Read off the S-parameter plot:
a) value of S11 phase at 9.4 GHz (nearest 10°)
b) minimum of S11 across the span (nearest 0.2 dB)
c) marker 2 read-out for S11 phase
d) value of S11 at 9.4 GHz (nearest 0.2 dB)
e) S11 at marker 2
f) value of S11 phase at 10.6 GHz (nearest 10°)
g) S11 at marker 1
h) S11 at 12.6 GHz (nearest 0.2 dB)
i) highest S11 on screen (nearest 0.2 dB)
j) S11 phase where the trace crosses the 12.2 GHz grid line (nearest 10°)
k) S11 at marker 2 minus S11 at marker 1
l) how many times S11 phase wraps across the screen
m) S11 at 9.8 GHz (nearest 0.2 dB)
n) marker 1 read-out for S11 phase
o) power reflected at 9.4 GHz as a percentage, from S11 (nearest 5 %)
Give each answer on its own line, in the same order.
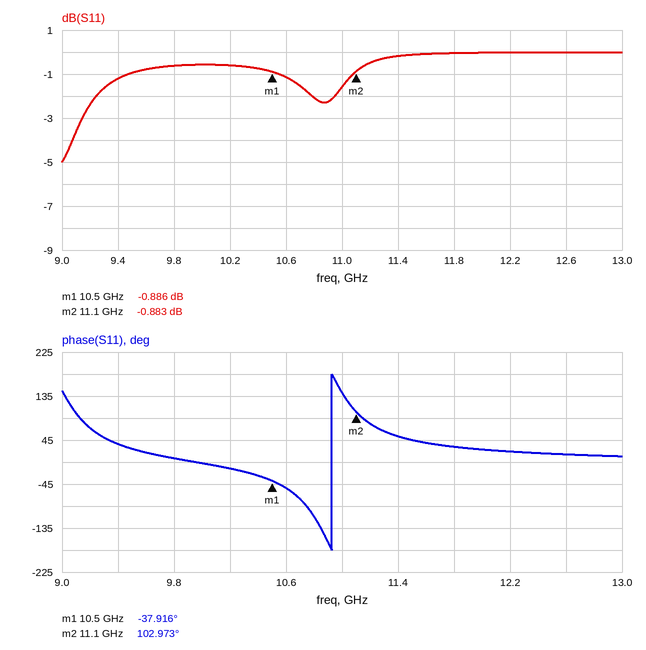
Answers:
40°
-5.0 dB
102.973°
-1.2 dB
-0.883 dB
-50°
-0.886 dB
0.0 dB
0.0 dB
20°
0.003 dB
1
-0.6 dB
-37.916°
75 %
